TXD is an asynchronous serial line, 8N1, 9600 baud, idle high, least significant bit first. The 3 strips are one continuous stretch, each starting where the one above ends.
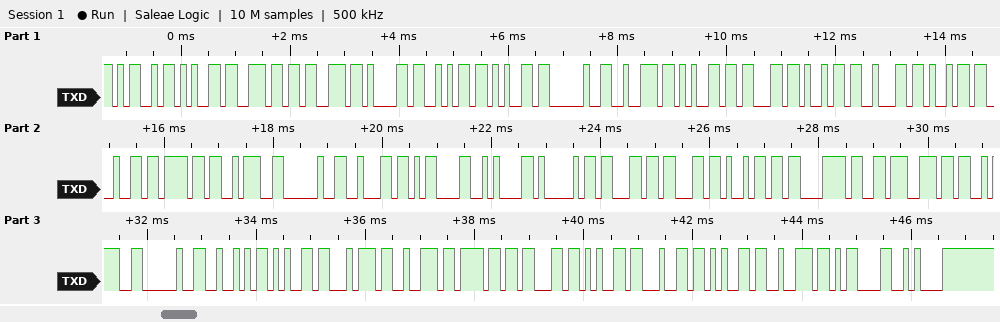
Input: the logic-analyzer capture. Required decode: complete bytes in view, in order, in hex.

0x4D 0x65 0x6E 0x73 0x61 0x6A 0x65 0x20 0x72 0x65 0x63 0x69 0x62 0x69 0x64 0x6F 0x3A 0x20 0x62 0x0D 0x0A 0x41 0x63 0x63 0x69 0xC3 0xB3 0x6E 0x3A 0x20 0x52 0x65 0x74 0x72 0x6F 0x63 0x65 0x64 0x65 0x72 0x0D 0x0A
